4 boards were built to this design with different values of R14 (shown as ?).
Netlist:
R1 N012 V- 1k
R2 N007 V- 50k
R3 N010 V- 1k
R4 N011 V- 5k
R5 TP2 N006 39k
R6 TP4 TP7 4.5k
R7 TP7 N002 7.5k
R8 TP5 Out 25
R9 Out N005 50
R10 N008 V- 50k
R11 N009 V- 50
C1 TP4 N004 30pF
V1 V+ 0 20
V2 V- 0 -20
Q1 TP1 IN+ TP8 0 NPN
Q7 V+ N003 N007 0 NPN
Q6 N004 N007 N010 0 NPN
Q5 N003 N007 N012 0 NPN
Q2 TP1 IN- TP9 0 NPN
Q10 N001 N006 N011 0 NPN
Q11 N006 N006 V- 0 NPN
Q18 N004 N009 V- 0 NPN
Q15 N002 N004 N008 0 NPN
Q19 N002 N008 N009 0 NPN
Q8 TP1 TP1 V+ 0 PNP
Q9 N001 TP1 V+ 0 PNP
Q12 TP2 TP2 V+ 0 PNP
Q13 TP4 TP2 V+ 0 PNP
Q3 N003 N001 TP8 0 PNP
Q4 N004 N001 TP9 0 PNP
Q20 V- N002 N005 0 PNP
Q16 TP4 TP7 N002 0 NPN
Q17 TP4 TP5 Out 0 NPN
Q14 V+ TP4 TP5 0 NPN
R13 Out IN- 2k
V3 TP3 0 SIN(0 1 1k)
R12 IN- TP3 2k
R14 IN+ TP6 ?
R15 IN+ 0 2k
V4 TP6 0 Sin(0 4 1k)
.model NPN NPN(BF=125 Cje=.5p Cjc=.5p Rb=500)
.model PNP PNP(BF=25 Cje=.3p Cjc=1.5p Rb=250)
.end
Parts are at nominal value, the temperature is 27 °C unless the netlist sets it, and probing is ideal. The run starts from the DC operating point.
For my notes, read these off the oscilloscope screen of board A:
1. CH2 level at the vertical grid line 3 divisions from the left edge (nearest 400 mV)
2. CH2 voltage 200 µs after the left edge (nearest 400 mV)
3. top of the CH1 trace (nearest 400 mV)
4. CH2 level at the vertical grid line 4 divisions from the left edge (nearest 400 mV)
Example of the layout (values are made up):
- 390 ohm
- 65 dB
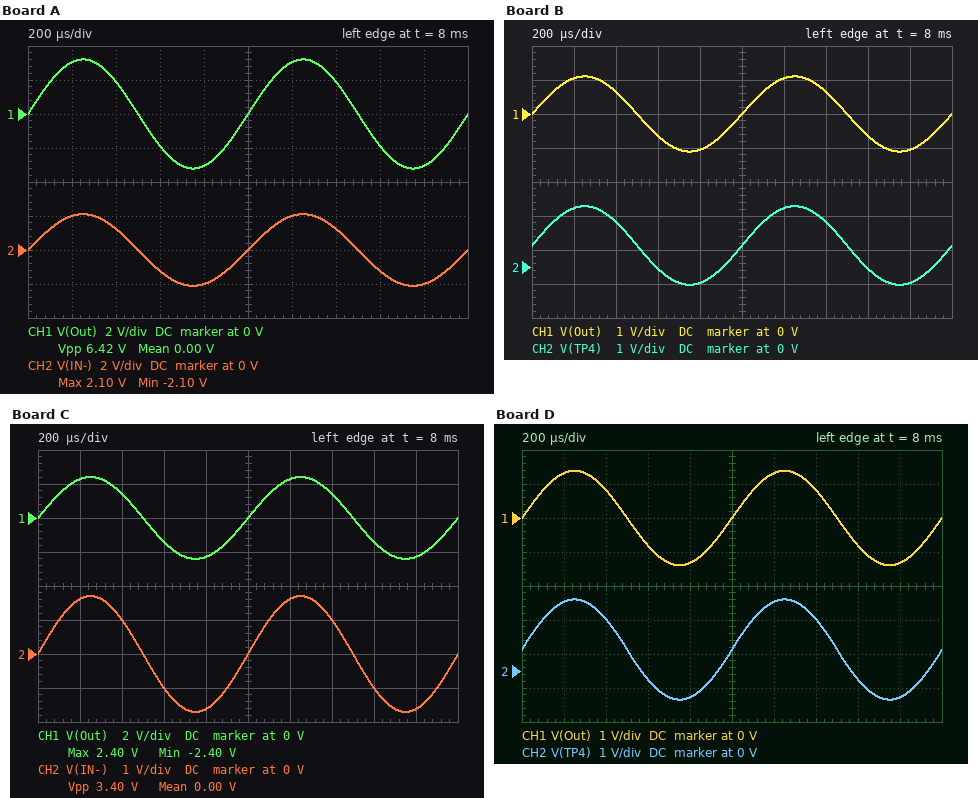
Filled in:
- -1.2 V
- 2.0 V
- 3.2 V
- -2.0 V
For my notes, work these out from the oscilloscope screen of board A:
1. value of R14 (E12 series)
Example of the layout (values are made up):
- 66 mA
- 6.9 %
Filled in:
- 1.8 kΩ
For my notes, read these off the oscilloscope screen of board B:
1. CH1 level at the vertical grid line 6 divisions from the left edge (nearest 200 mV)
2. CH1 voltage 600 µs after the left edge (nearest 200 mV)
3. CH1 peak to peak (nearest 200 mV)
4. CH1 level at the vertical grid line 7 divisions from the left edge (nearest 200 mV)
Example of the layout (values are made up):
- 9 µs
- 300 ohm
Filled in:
- 1.0 V
- -600 mV
- 2.2 V
- 600 mV
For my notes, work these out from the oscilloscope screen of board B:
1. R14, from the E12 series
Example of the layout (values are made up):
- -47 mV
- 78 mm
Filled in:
- 5.6 kΩ
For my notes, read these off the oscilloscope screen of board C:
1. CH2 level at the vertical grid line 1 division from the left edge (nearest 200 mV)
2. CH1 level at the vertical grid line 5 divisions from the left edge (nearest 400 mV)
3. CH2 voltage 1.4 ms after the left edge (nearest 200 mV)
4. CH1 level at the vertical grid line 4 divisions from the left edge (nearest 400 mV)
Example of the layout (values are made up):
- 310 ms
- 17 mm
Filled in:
- 1.6 V
- 0 V
- 1.0 V
- -2.4 V
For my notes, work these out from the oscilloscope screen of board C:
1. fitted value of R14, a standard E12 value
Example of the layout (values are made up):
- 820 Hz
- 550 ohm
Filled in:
- 2.7 kΩ
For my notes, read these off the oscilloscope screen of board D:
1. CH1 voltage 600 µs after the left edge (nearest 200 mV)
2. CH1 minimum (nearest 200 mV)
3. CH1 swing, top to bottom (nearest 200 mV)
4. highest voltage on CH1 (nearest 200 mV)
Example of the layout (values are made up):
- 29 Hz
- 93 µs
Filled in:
- -800 mV
- -1.4 V
- 2.8 V
- 1.4 V
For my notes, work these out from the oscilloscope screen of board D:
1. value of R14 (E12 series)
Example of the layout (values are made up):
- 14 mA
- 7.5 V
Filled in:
- 4.7 kΩ
